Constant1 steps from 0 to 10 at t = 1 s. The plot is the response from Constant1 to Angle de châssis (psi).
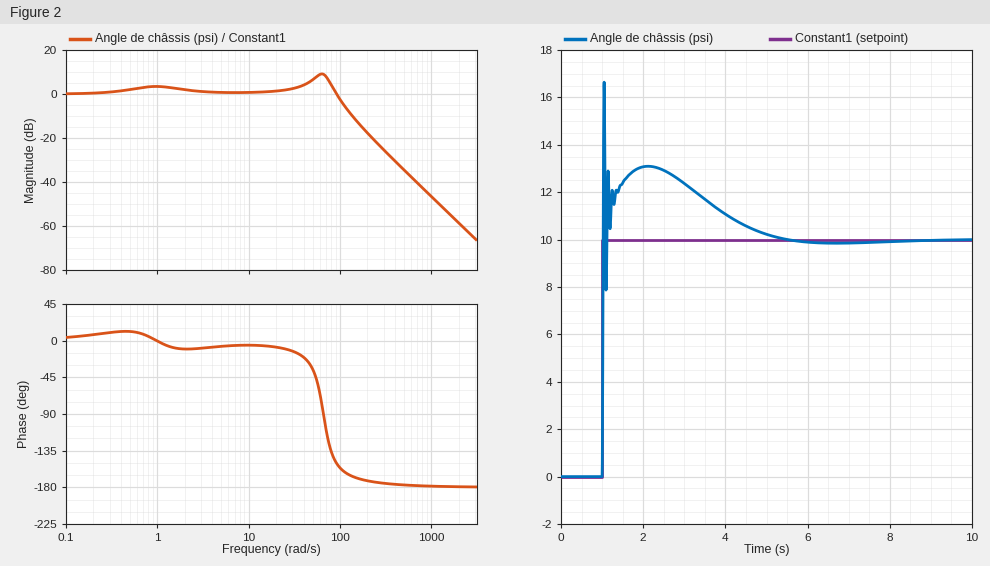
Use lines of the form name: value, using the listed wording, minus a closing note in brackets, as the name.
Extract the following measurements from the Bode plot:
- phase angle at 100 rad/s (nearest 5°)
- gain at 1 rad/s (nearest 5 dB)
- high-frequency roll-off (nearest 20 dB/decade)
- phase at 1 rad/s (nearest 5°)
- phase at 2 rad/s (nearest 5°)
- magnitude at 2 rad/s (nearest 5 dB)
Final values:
phase angle at 100 rad/s: -155°
gain at 1 rad/s: 5 dB
high-frequency roll-off: -40 dB/decade
phase at 1 rad/s: 0°
phase at 2 rad/s: -10°
magnitude at 2 rad/s: 0 dB
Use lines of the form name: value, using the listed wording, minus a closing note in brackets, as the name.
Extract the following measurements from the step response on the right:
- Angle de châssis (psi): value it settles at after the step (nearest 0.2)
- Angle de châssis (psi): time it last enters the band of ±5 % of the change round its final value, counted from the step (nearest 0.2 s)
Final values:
Angle de châssis (psi): value it settles at after the step: 10.0
Angle de châssis (psi): time it last enters the band of ±5 % of the change round its final value, counted from the step: 3.6 s
